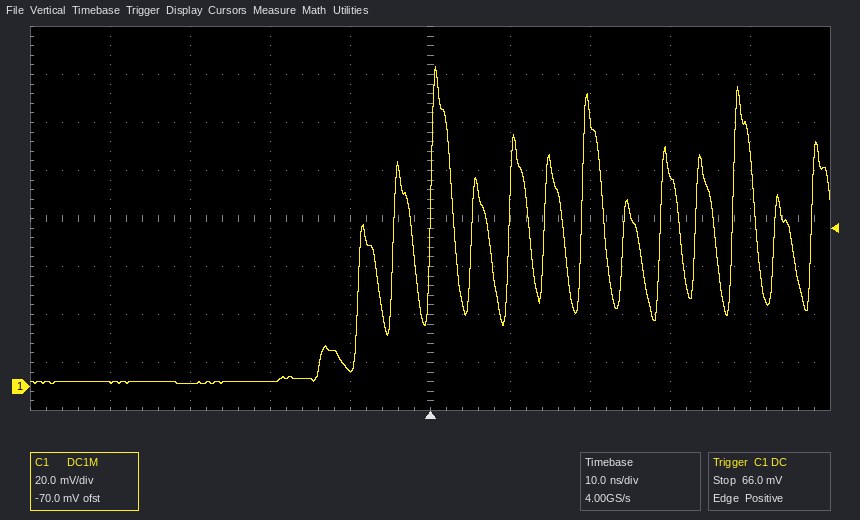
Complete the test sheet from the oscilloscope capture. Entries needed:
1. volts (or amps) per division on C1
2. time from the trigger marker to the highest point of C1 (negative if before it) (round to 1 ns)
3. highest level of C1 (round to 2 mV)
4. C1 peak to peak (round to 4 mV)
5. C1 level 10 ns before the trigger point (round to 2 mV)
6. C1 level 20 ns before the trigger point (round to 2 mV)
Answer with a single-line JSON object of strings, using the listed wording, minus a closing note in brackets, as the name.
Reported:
{"volts (or amps) per division on C1": "20 mV", "time from the trigger marker to the highest point of C1 (negative if before it)": "+1 ns", "highest level of C1": "134 mV", "C1 peak to peak": "132 mV", "C1 level 10 ns before the trigger point": "8 mV", "C1 level 20 ns before the trigger point": "2 mV"}
